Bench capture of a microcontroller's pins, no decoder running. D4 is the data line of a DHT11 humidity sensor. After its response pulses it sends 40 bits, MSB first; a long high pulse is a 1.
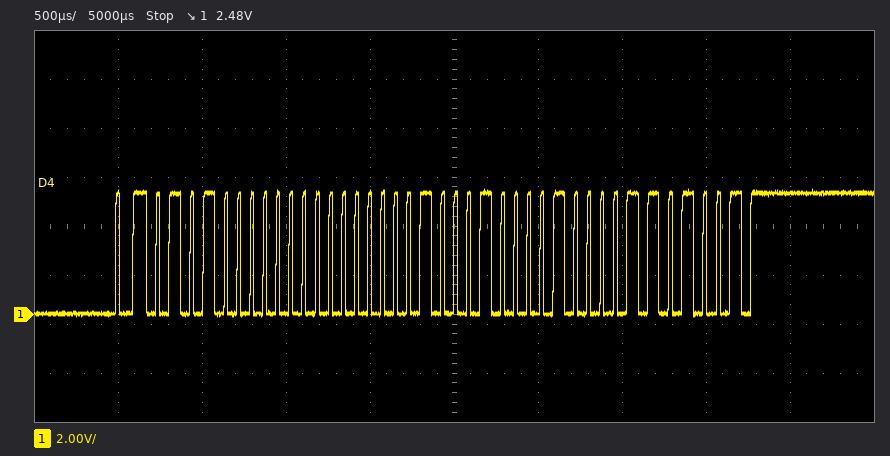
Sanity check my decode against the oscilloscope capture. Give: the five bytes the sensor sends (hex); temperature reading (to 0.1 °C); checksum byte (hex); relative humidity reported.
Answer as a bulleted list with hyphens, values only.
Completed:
- 50 00 11 08 69
- 17.8 °C
- 0x69
- 80 %
